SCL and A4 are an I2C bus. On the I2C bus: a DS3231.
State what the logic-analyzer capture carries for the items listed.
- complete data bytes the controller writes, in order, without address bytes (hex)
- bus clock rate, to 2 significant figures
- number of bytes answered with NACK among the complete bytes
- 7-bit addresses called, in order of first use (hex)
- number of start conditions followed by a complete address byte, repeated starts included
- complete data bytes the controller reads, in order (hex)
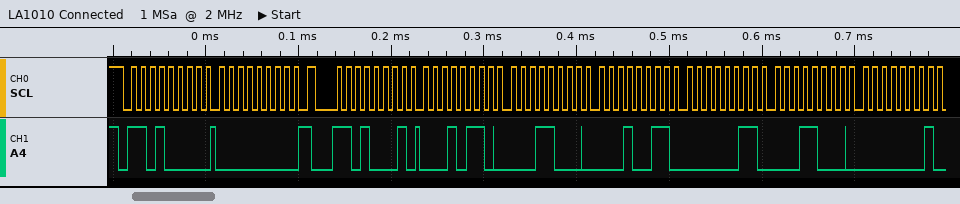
00
100 kHz
0
0x68
2
16 18 13 03 18 01
